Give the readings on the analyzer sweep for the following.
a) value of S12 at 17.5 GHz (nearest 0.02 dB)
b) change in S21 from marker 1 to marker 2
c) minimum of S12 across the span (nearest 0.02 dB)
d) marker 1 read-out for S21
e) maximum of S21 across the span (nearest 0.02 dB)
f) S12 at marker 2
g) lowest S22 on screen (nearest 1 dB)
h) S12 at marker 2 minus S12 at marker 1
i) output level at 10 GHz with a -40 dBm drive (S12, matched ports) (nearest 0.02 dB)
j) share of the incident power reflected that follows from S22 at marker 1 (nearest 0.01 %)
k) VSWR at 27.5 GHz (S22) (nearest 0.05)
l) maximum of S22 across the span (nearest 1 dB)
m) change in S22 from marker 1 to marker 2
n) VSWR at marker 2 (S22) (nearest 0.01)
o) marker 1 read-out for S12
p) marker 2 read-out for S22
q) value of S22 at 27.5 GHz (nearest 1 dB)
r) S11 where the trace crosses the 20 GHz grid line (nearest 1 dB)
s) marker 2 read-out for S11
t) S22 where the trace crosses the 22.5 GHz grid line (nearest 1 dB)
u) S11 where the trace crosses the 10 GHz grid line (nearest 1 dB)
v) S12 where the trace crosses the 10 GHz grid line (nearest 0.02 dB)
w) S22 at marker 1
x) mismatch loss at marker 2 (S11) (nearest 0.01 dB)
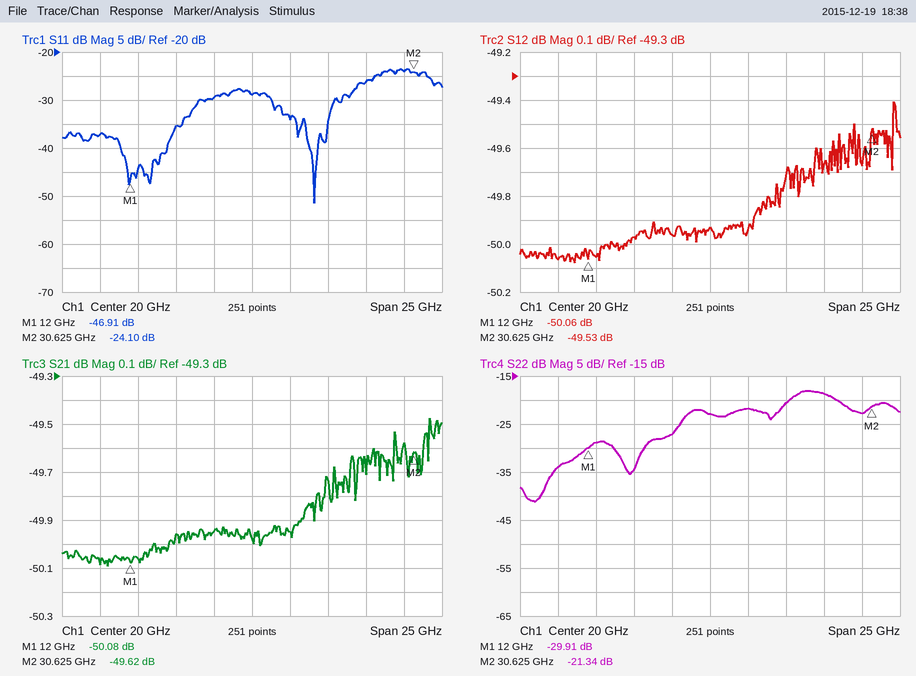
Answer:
-49.96 dB
0.46 dB
-50.08 dB
-50.08 dB
-49.48 dB
-49.53 dB
-41 dB
0.53 dB
-90.06 dBm
0.10 %
1.25
-18 dB
8.57 dB
1.19
-50.06 dB
-21.34 dB
-19 dB
-29 dB
-24.10 dB
-22 dB
-37 dB
-50.06 dB
-29.91 dB
0.02 dB
